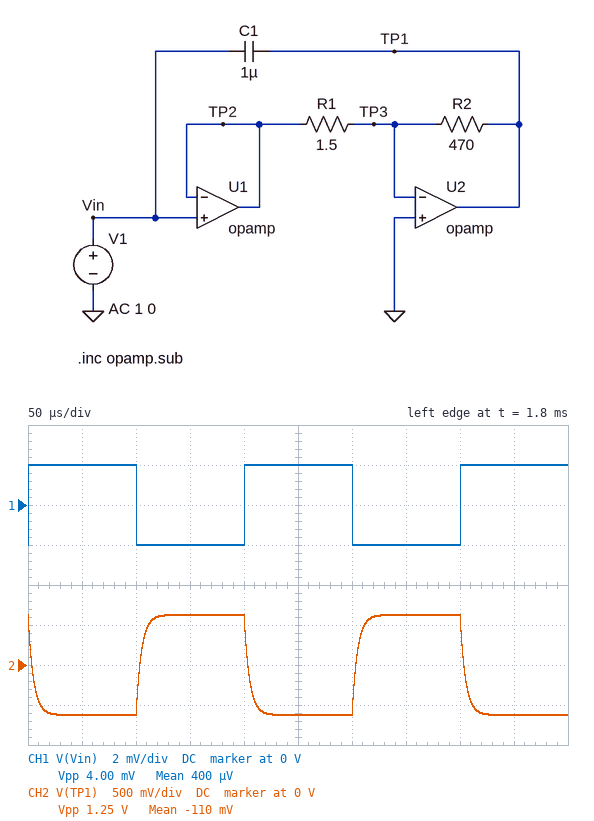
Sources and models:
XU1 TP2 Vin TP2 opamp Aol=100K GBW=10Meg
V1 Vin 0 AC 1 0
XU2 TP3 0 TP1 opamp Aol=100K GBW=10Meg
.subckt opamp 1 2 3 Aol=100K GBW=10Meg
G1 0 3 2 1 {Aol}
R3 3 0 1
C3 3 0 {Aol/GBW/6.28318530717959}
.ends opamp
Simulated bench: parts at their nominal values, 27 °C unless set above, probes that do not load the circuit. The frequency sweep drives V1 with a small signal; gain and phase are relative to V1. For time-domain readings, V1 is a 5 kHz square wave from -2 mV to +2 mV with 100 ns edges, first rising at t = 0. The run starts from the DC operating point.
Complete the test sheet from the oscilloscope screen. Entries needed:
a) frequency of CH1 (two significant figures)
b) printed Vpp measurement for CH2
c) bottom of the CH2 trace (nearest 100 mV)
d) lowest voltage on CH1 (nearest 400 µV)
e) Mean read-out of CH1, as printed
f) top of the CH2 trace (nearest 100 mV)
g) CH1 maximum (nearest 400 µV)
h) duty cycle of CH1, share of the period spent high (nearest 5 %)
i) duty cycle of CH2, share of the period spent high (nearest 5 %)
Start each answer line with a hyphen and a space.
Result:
- 5.0 kHz
- 1.25 V
- -600 mV
- -2.0 mV
- 400 µV
- 600 mV
- 2.0 mV
- 50 %
- 50 %
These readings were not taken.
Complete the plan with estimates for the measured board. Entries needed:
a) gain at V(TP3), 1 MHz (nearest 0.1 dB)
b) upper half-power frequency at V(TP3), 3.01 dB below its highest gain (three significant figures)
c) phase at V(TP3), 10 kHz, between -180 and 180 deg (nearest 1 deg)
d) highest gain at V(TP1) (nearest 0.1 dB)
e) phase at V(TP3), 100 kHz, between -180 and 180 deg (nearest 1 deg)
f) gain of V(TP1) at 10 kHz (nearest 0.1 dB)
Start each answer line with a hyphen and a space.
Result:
- -0.1 dB
- 10.1 MHz
- 72 deg
- 49.9 dB
- 17 deg
- 49.5 dB
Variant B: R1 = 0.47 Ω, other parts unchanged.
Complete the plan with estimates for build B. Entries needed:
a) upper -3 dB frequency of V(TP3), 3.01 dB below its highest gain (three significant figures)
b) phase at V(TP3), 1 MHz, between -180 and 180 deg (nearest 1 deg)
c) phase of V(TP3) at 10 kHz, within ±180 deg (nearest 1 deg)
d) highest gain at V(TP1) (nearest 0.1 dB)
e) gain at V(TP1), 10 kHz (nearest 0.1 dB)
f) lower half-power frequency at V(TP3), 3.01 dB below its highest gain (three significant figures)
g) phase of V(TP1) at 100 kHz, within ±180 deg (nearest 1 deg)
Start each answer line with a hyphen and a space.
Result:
- 10.0 MHz
- -5 deg
- 45 deg
- 59.9 dB
- 56.9 dB
- 10.1 kHz
- 95 deg
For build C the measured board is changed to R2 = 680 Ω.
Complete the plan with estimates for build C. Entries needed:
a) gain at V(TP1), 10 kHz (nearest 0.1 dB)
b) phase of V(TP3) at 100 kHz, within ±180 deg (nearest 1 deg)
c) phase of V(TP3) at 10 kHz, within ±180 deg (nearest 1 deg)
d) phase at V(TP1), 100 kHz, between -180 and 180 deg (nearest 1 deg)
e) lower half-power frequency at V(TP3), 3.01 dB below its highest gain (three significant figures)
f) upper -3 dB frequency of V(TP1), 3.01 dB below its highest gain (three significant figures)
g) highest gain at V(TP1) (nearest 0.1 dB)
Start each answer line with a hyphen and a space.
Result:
- 52.3 dB
- 12 deg
- 65 deg
- 102 deg
- 22.0 kHz
- 22.1 kHz
- 53.1 dB
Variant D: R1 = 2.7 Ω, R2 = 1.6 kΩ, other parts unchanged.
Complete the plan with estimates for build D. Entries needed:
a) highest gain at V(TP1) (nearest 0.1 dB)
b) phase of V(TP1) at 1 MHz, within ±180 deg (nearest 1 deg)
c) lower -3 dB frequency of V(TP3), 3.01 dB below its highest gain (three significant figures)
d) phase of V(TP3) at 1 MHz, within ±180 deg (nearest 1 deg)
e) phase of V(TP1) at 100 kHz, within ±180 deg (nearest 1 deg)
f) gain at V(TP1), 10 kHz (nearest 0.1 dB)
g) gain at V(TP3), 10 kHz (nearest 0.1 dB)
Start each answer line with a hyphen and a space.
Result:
- 55.4 dB
- 85 deg
- 16.9 kHz
- -5 deg
- 99 deg
- 54.1 dB
- -5.9 dB
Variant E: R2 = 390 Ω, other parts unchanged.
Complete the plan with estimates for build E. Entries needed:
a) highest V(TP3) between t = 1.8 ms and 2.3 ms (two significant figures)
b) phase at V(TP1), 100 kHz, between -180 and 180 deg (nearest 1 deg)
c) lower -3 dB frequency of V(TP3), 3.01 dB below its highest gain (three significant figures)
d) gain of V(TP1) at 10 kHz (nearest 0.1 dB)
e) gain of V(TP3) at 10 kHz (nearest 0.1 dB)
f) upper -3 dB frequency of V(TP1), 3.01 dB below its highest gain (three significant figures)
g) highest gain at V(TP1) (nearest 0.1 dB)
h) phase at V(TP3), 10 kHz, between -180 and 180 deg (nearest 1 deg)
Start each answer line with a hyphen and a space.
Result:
- 3.9 mV
- 110 deg
- 38.1 kHz
- 48.0 dB
- -12.0 dB
- 38.4 kHz
- 48.3 dB
- 75 deg
